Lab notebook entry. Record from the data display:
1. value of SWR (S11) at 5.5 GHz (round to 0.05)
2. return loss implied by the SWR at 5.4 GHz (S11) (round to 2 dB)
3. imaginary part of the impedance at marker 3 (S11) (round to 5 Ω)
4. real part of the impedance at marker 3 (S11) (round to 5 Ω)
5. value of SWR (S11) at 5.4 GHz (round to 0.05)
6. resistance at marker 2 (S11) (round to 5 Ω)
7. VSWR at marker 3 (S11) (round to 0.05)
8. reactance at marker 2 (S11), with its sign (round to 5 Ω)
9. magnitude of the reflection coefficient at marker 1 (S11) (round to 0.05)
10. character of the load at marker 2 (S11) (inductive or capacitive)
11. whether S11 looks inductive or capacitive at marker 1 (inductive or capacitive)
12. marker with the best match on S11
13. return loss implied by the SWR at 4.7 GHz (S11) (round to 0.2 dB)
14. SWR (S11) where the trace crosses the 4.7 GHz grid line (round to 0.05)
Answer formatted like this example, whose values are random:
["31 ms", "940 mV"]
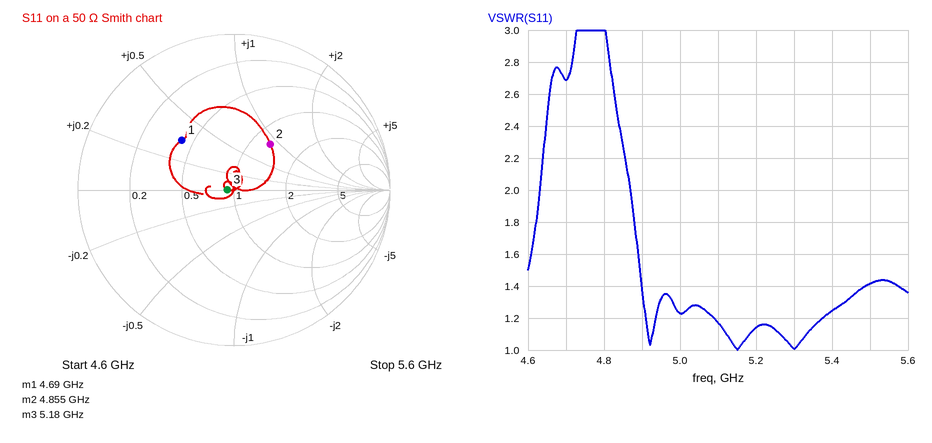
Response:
["1.40", "20 dB", "0 Ω", "45 Ω", "1.25", "65 Ω", "1.10", "+45 Ω", "0.45", "inductive", "inductive", "marker 3", "6.8 dB", "2.70"]
